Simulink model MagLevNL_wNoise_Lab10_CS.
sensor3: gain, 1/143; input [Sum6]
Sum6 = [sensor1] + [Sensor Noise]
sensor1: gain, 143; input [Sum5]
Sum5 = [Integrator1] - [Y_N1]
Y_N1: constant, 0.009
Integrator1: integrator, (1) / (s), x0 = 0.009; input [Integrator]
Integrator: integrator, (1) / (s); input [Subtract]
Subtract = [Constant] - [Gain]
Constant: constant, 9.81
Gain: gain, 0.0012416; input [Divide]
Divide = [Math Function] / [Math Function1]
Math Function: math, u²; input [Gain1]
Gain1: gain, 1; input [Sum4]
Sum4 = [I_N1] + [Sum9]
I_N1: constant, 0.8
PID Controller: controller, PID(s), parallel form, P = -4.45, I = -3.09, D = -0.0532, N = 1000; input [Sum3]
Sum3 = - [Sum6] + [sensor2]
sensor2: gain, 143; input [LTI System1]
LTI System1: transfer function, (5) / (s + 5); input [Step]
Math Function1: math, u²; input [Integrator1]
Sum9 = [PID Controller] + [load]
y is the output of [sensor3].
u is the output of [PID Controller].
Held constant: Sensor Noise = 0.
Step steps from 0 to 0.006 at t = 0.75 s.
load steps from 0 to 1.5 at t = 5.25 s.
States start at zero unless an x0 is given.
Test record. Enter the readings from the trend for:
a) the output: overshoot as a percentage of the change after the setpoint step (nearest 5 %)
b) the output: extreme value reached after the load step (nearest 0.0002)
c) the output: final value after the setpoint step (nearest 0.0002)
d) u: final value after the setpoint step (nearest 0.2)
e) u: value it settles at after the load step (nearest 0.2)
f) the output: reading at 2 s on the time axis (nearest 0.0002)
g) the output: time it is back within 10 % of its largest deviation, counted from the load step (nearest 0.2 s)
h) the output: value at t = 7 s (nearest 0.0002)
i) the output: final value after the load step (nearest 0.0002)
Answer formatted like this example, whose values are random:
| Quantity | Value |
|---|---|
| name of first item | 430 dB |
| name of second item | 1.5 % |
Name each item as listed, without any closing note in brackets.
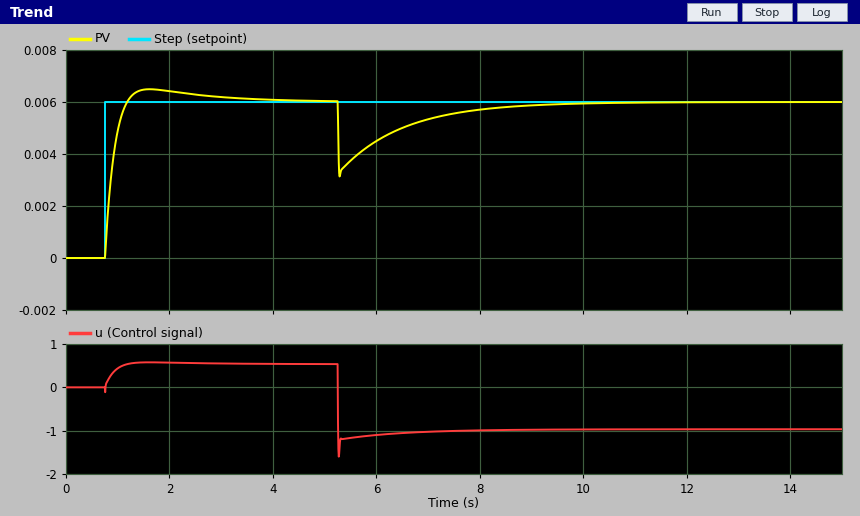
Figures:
| Quantity | Value |
|---|---|
| the output: overshoot as a percentage of the change after the setpoint step | 10 % |
| the output: extreme value reached after the load step | 0.0032 |
| the output: final value after the setpoint step | 0.0060 |
| u: final value after the setpoint step | 0.6 |
| u: value it settles at after the load step | -1.0 |
| the output: reading at 2 s on the time axis | 0.0064 |
| the output: time it is back within 10 % of its largest deviation, counted from the load step | 2.8 s |
| the output: value at t = 7 s | 0.0054 |
| the output: final value after the load step | 0.0060 |
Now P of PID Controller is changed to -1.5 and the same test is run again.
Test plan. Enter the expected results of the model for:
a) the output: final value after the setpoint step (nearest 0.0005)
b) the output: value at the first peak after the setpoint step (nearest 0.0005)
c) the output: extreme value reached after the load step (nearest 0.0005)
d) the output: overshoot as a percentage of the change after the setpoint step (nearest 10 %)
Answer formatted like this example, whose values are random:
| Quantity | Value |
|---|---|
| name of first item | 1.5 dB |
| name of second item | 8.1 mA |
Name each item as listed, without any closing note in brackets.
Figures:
| Quantity | Value |
|---|---|
| the output: final value after the setpoint step | 0.0060 |
| the output: value at the first peak after the setpoint step | 0.0070 |
| the output: extreme value reached after the load step | -0.0030 |
| the output: overshoot as a percentage of the change after the setpoint step | 20 % |
